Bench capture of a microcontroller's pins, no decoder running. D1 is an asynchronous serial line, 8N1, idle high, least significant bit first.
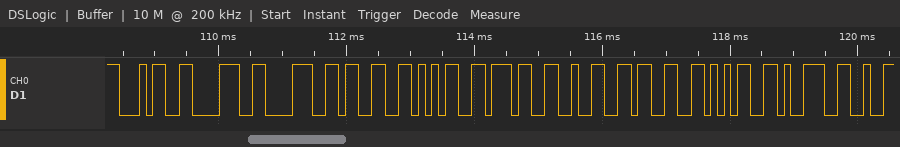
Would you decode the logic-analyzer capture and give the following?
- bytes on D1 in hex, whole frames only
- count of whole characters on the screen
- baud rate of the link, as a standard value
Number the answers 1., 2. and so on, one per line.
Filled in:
1. 0x34 0x38 0x38 0x33 0x35 0x37 0x32 0x33 0x35 0x39
2. 10
3. 9600 baud
